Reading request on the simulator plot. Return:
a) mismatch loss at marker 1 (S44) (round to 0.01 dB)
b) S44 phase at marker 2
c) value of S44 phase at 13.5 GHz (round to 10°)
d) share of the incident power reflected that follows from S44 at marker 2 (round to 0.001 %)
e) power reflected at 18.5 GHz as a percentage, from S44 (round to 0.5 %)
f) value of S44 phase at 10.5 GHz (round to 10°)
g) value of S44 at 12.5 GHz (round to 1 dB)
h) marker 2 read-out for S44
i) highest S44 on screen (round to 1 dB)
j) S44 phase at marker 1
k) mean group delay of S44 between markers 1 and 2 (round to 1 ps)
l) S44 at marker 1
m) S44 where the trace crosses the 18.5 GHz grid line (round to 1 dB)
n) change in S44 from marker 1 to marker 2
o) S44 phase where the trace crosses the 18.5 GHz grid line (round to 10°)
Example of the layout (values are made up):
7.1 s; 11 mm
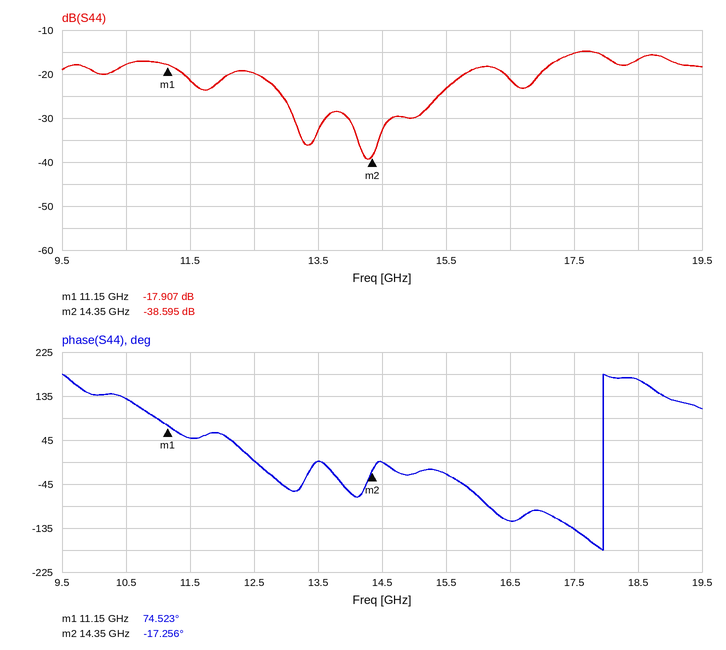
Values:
0.07 dB; -17.256°; 0°; 0.014 %; 2.0 %; 130°; -20 dB; -38.595 dB; -15 dB; 74.523°; 80 ps; -17.907 dB; -17 dB; -20.688 dB; 170°
